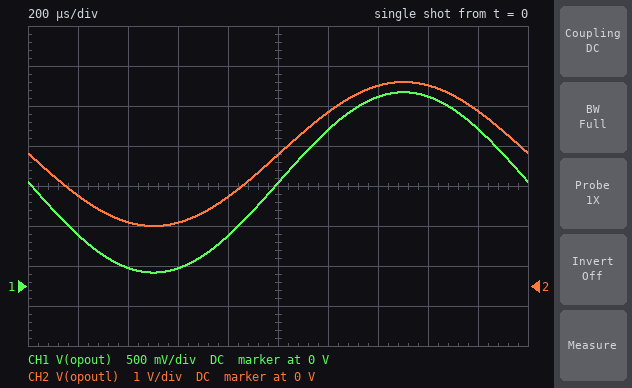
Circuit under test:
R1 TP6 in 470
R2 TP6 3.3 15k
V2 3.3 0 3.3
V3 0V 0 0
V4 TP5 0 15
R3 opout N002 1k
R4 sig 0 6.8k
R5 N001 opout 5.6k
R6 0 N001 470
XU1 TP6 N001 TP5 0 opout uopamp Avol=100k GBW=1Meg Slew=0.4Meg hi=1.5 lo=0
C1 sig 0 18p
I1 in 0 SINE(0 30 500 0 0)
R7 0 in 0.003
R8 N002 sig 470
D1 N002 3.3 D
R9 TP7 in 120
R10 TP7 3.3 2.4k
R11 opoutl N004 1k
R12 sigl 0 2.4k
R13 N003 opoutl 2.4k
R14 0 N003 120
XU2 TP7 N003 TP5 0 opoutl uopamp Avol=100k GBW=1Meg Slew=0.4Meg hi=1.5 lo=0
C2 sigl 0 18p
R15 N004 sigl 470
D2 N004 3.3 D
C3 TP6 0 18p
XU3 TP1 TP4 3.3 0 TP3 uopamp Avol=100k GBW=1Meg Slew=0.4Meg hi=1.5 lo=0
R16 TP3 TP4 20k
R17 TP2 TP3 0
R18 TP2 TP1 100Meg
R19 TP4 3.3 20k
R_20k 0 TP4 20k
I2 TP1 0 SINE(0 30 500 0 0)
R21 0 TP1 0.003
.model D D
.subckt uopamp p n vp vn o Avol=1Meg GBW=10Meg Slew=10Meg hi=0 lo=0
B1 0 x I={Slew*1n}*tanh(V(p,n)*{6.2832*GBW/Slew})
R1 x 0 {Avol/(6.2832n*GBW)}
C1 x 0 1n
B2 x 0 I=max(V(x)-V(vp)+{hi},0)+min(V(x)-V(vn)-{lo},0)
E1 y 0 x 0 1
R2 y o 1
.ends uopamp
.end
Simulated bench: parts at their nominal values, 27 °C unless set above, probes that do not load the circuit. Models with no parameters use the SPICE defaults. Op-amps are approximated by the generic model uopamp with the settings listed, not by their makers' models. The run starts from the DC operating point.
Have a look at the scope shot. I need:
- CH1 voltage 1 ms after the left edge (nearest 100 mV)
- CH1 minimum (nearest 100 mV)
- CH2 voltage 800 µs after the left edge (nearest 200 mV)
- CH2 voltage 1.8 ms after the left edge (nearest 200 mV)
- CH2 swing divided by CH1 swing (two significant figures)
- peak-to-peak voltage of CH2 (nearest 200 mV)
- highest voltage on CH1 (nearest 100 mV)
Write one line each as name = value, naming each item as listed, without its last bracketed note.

CH1 voltage 1 ms after the left edge = 1.3 V
CH1 minimum = 200 mV
CH2 voltage 800 µs after the left edge = 2.2 V
CH2 voltage 1.8 ms after the left edge = 4.4 V
CH2 swing divided by CH1 swing = 1.6
peak-to-peak voltage of CH2 = 3.6 V
highest voltage on CH1 = 2.4 V
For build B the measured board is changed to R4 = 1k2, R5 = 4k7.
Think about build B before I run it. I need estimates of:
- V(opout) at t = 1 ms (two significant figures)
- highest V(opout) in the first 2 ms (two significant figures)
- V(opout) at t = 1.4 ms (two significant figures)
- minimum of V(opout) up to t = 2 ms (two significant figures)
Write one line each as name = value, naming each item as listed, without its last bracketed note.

V(opout) at t = 1 ms = 1.1 V
highest V(opout) in the first 2 ms = 2.1 V
V(opout) at t = 1.4 ms = 2.0 V
minimum of V(opout) up to t = 2 ms = 140 mV
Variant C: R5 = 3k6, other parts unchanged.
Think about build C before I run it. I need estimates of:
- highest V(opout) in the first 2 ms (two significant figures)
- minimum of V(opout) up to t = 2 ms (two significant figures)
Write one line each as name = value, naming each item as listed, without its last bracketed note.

highest V(opout) in the first 2 ms = 1.6 V
minimum of V(opout) up to t = 2 ms = 110 mV
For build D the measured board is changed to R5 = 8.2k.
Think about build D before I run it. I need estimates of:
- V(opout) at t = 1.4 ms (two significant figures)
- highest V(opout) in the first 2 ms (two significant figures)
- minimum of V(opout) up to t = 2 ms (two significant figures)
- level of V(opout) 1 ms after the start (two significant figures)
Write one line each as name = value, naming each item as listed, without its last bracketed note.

V(opout) at t = 1.4 ms = 3.4 V
highest V(opout) in the first 2 ms = 3.5 V
minimum of V(opout) up to t = 2 ms = 240 mV
level of V(opout) 1 ms after the start = 1.8 V
